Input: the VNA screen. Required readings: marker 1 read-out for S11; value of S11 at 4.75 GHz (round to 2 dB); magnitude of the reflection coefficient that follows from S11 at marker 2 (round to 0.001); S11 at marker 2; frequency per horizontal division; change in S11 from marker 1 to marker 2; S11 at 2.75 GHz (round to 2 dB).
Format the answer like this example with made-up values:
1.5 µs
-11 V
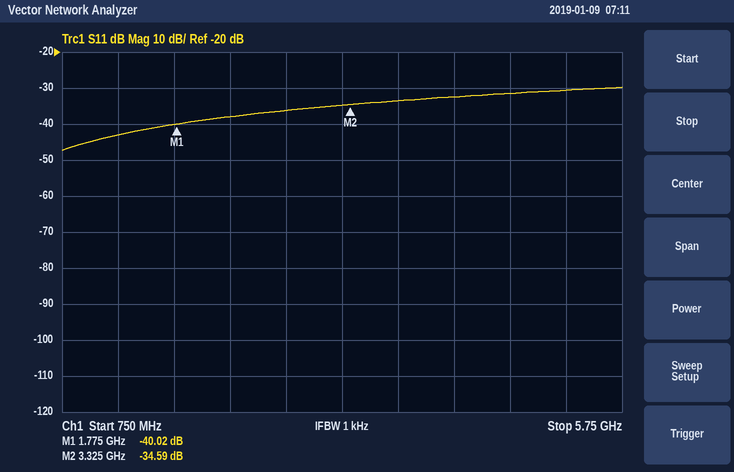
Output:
-40.02 dB
-32 dB
0.019
-34.59 dB
500 MHz
5.43 dB
-36 dB
